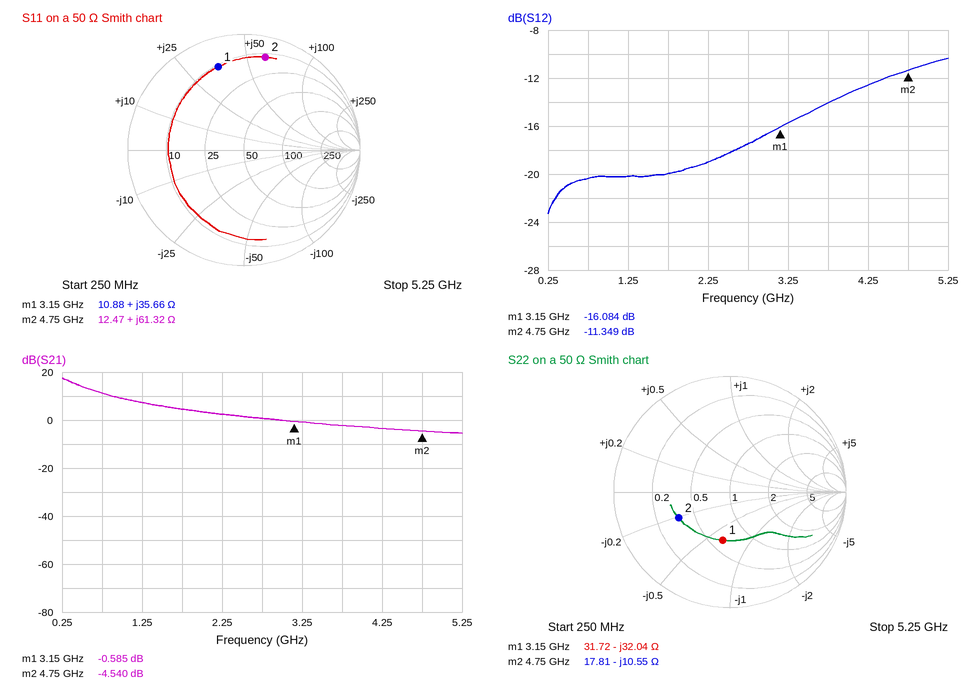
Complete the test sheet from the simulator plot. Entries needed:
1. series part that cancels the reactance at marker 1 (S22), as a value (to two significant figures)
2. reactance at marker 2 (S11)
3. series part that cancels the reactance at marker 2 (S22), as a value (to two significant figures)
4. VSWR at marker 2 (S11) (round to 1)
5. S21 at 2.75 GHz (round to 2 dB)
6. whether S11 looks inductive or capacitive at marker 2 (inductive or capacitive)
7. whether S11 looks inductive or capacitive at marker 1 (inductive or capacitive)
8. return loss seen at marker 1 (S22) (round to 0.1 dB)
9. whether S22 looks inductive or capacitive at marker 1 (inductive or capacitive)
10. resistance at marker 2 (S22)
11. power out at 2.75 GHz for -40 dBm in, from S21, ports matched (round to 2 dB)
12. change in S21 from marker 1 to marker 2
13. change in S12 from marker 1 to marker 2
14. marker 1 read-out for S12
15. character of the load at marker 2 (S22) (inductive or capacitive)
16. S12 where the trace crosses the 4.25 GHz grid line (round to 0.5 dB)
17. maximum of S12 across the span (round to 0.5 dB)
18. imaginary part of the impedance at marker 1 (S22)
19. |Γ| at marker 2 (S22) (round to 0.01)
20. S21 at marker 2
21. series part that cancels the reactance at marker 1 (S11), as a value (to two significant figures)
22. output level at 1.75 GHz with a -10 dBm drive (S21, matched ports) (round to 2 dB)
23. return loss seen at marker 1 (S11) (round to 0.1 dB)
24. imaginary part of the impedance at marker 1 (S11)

1.6 nH
+61.32 Ω
350 pH
10
0 dB
inductive
inductive
7.5 dB
capacitive
17.81 Ω
-40 dBm
-3.955 dB
4.735 dB
-16.084 dB
capacitive
-12.5 dB
-10.5 dB
-32.04 Ω
0.49
-4.540 dB
1.4 pF
-6 dBm
2.5 dB
+35.66 Ω
